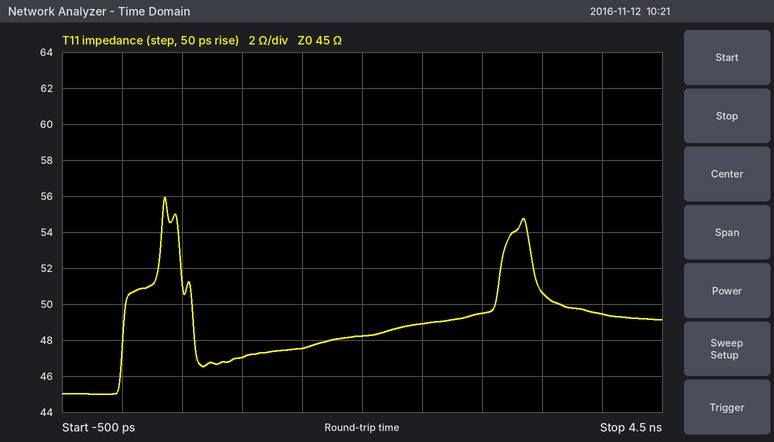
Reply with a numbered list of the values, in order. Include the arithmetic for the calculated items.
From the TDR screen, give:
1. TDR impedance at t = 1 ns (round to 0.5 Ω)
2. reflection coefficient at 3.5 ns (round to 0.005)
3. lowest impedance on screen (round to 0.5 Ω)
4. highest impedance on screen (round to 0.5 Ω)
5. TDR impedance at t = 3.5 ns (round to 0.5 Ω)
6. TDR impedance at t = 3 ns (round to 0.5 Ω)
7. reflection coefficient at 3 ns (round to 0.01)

1. 47.0 Ω
2. (50.5 − 45)/(50.5 + 45) ≈ +0.0576, so +0.060 to the nearest 0.005
3. 45.0 Ω
4. 56.0 Ω
5. 50.5 Ω
6. 49.5 Ω
7. (49.5 − 45)/(49.5 + 45) ≈ +0.05
